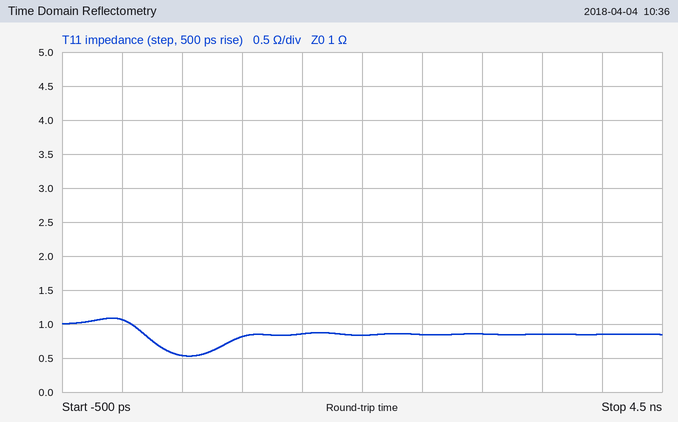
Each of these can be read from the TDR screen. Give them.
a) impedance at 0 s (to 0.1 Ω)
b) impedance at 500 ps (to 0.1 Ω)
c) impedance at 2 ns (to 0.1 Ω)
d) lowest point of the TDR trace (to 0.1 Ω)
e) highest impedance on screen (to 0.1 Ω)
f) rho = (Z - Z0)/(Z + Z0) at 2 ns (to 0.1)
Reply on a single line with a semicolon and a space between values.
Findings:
1.1 Ω; 0.5 Ω; 0.8 Ω; 0.5 Ω; 1.1 Ω; -0.1
